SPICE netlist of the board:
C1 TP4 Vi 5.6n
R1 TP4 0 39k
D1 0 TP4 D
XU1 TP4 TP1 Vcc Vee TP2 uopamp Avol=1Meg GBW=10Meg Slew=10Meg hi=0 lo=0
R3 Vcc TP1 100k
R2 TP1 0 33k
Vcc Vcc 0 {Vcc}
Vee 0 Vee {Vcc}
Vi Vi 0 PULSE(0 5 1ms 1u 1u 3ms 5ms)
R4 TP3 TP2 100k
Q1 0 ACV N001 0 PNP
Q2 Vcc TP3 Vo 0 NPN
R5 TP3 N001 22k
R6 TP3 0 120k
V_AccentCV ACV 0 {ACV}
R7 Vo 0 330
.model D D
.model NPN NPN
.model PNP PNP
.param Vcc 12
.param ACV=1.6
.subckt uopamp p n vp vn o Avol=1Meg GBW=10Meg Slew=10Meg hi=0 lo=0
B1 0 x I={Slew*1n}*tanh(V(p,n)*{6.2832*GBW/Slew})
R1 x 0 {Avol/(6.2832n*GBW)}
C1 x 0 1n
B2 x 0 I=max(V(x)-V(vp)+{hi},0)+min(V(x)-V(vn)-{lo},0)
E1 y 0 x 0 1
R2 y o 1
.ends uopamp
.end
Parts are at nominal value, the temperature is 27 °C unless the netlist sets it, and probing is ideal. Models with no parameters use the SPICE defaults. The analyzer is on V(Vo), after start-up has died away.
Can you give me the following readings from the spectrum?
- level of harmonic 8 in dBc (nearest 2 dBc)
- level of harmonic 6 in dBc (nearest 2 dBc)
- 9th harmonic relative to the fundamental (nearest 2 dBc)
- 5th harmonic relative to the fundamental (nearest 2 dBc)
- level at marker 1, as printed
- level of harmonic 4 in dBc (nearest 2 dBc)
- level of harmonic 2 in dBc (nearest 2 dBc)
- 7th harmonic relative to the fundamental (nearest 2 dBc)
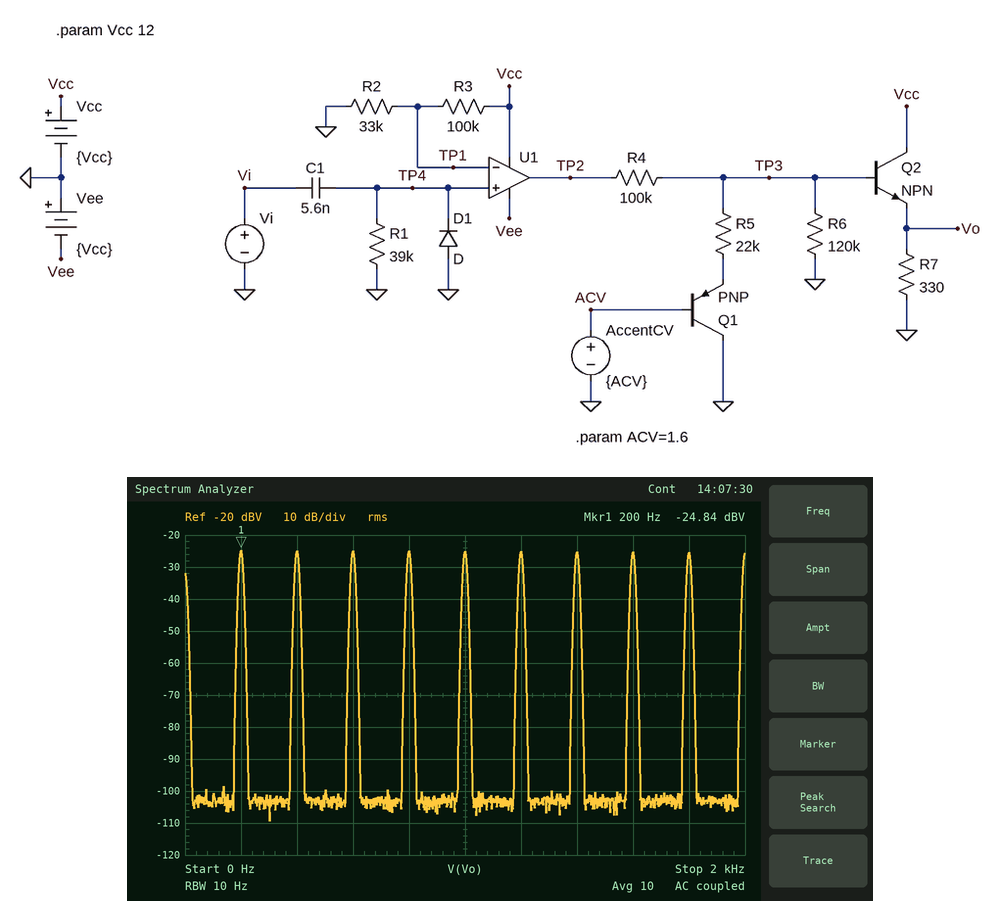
0 dBc
0 dBc
0 dBc
0 dBc
-24.84 dBV
0 dBc
0 dBc
0 dBc
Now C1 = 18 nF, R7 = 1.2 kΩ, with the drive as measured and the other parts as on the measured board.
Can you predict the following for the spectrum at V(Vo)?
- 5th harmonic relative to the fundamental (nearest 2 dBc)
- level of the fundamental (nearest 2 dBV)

-2 dBc
-12 dBV
